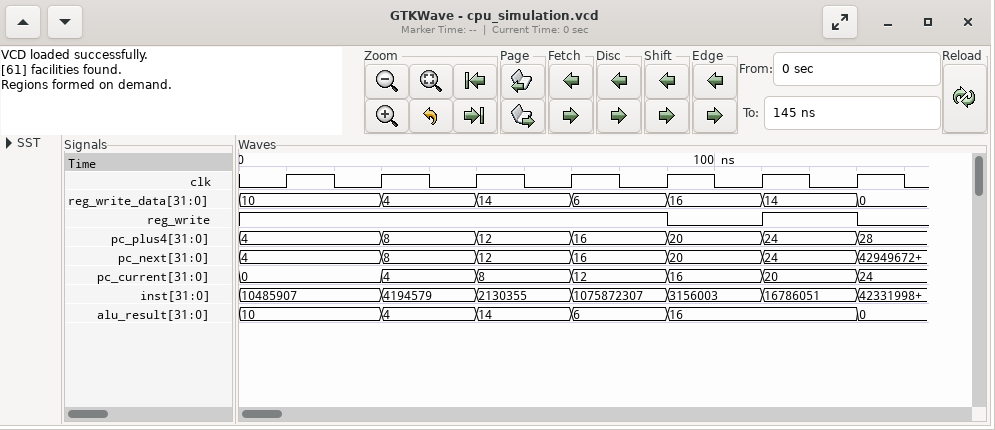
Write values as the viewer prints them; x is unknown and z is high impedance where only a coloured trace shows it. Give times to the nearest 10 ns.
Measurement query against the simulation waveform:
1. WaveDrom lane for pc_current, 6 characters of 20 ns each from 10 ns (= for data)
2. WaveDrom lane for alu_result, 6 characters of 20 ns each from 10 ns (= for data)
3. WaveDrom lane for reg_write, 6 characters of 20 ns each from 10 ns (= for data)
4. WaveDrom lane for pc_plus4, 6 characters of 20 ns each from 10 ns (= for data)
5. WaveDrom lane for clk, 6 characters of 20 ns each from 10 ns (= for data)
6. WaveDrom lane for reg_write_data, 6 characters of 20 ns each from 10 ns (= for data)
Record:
{name: 'pc_current', wave: '======', data: '0 4 8 12 16 20'}
{name: 'alu_result', wave: '=====.', data: '10 4 14 6 16'}
{name: 'reg_write', wave: '1...01'}
{name: 'pc_plus4', wave: '======', data: '4 8 12 16 20 24'}
{name: 'clk', wave: 'p.....'}
{name: 'reg_write_data', wave: '======', data: '10 4 14 6 16 14'}
